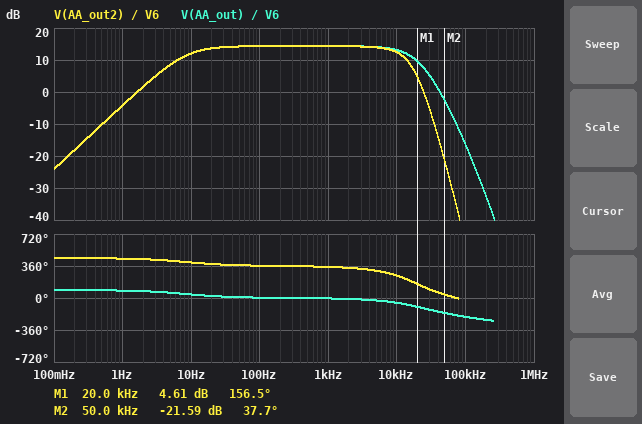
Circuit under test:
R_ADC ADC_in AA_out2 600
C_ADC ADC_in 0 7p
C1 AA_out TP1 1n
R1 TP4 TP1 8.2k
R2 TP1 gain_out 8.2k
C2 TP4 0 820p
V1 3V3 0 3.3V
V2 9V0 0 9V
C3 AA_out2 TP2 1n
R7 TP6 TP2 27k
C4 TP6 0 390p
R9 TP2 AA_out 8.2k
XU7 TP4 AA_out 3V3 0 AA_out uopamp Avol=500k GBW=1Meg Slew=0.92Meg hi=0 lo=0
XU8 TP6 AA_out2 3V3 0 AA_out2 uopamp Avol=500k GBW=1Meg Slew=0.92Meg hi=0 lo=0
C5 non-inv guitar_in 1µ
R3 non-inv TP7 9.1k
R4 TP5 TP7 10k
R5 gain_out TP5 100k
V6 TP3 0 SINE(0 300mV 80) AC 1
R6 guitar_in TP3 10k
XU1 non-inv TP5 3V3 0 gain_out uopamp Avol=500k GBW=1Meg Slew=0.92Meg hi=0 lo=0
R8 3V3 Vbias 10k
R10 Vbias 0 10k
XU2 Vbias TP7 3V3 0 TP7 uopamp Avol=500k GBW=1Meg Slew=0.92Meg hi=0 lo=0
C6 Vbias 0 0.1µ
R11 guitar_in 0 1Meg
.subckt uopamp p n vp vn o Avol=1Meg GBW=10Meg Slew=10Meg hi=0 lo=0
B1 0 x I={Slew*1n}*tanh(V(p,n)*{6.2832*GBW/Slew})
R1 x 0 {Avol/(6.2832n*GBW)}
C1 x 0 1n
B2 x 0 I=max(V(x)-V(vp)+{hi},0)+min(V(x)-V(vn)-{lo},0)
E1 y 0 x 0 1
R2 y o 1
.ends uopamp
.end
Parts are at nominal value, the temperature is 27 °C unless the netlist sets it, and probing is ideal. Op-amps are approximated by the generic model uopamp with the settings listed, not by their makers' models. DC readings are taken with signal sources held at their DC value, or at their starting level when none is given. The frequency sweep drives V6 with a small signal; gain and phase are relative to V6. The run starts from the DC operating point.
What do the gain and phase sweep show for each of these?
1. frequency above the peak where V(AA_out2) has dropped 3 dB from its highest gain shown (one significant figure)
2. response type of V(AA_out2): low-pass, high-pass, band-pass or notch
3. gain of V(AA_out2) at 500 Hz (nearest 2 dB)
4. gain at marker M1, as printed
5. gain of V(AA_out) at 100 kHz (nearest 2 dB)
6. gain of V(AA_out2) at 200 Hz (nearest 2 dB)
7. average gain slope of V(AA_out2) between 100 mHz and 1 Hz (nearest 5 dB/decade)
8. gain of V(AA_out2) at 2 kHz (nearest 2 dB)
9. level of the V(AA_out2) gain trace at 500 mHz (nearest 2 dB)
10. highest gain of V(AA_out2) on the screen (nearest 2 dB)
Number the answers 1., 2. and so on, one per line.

1. 10 kHz
2. band-pass
3. 14 dB
4. 4.61 dB
5. -16 dB
6. 14 dB
7. 20 dB/decade
8. 14 dB
9. -10 dB
10. 14 dB
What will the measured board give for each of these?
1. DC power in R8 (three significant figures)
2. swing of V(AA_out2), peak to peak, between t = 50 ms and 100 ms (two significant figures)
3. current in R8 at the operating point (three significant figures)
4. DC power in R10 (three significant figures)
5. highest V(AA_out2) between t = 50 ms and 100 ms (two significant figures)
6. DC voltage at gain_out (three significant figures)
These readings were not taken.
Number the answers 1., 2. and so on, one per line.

1. 272 µW
2. 3.1 V
3. 165 µA
4. 272 µW
5. 3.2 V
6. 1.65 V
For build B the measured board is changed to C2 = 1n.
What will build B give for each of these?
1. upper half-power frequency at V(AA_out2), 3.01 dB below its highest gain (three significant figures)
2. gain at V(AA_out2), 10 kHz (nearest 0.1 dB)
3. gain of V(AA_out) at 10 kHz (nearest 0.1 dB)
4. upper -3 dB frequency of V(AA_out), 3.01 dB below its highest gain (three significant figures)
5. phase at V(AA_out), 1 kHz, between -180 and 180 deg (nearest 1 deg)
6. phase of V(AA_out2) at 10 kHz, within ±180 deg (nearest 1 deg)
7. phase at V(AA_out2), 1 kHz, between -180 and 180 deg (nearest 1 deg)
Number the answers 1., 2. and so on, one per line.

1. 10.4 kHz
2. 11.6 dB
3. 12.3 dB
4. 12.4 kHz
5. -6 deg
6. -115 deg
7. -11 deg
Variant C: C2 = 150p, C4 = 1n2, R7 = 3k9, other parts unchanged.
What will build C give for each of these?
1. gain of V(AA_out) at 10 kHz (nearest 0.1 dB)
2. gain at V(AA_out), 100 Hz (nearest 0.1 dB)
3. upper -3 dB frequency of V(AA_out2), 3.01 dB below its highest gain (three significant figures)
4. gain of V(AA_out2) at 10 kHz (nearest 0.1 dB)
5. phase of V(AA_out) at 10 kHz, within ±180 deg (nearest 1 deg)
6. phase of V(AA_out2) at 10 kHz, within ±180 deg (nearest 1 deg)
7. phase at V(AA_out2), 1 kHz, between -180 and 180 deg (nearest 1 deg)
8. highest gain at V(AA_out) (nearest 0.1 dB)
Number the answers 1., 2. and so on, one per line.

1. 14.6 dB
2. 14.3 dB
3. 14.8 kHz
4. 12.7 dB
5. -16 deg
6. -64 deg
7. -6 deg
8. 16.9 dB
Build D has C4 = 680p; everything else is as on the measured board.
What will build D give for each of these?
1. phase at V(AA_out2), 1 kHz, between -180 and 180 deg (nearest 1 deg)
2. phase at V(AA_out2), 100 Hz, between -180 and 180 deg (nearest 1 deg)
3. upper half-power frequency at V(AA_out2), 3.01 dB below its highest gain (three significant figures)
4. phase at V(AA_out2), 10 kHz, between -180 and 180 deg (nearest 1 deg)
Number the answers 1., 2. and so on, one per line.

1. -14 deg
2. 3 deg
3. 7.48 kHz
4. -130 deg
